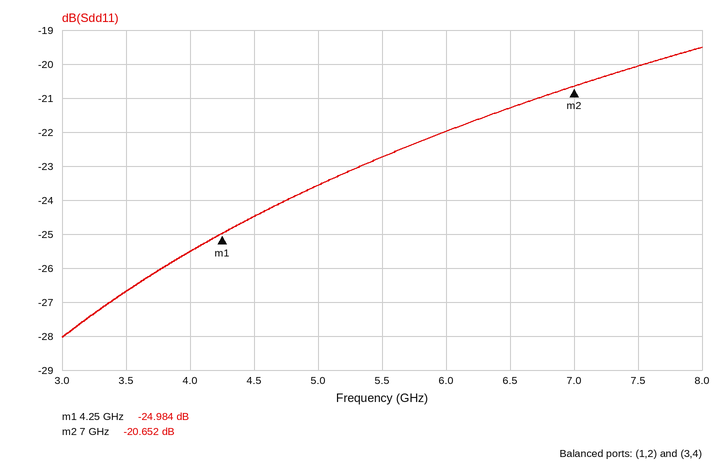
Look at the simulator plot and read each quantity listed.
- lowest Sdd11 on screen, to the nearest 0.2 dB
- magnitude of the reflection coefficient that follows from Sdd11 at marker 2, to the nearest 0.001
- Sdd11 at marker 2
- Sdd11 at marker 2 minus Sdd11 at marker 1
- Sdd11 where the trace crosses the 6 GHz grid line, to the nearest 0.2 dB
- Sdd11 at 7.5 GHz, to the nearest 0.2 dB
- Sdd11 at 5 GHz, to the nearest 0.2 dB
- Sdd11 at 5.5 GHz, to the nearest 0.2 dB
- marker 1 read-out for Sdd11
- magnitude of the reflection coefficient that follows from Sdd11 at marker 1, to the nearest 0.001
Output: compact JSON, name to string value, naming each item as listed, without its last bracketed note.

{"lowest Sdd11 on screen, to the nearest 0.2 dB": "-28.0 dB", "magnitude of the reflection coefficient that follows from Sdd11 at marker 2, to the nearest 0.001": "0.093", "Sdd11 at marker 2": "-20.652 dB", "Sdd11 at marker 2 minus Sdd11 at marker 1": "4.332 dB", "Sdd11 where the trace crosses the 6 GHz grid line, to the nearest 0.2 dB": "-22.0 dB", "Sdd11 at 7.5 GHz, to the nearest 0.2 dB": "-20.0 dB", "Sdd11 at 5 GHz, to the nearest 0.2 dB": "-23.6 dB", "Sdd11 at 5.5 GHz, to the nearest 0.2 dB": "-22.8 dB", "marker 1 read-out for Sdd11": "-24.984 dB", "magnitude of the reflection coefficient that follows from Sdd11 at marker 1, to the nearest 0.001": "0.056"}
